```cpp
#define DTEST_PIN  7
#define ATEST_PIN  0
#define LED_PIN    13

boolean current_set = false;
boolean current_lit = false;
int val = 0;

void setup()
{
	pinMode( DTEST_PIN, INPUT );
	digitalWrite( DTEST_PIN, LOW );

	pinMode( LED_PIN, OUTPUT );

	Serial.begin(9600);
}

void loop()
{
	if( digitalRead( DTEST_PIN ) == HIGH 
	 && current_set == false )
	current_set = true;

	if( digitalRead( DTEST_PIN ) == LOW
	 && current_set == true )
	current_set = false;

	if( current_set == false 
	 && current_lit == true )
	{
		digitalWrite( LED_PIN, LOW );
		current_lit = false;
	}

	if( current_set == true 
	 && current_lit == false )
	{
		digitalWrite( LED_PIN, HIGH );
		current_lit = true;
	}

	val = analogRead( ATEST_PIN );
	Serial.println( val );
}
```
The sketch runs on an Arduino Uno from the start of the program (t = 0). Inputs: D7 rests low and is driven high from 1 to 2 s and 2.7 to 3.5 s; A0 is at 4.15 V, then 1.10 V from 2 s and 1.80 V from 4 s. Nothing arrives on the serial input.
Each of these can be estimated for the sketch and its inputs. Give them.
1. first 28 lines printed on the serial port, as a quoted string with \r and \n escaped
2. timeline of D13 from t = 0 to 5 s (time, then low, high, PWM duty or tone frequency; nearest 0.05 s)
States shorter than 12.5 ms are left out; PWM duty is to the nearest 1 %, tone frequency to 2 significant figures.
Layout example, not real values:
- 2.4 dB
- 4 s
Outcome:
- "849\r\n849\r\n849\r\n849\r\n849\r\n849\r\n849\r\n849\r\n849\r\n849\r\n849\r\n849\r\n849\r\n849\r\n849\r\n849\r\n849\r\n849\r\n849\r\n849\r\n849\r\n849\r\n849\r\n849\r\n849\r\n849\r\n849\r\n849\r\n"
- 0 s low; 1 s high; 2 s low; 2.7 s high; 3.5 s low
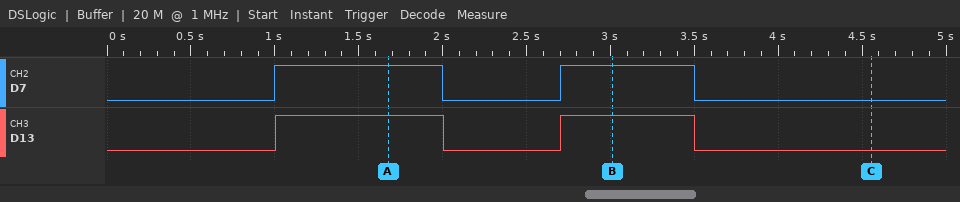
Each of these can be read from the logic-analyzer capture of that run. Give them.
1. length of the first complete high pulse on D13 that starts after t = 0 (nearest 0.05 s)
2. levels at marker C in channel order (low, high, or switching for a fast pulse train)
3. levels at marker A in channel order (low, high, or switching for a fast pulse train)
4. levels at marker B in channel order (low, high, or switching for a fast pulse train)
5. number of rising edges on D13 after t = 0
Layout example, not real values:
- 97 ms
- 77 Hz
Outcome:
- 1.00 s
- D7 low, D13 low
- D7 high, D13 high
- D7 high, D13 high
- 2
